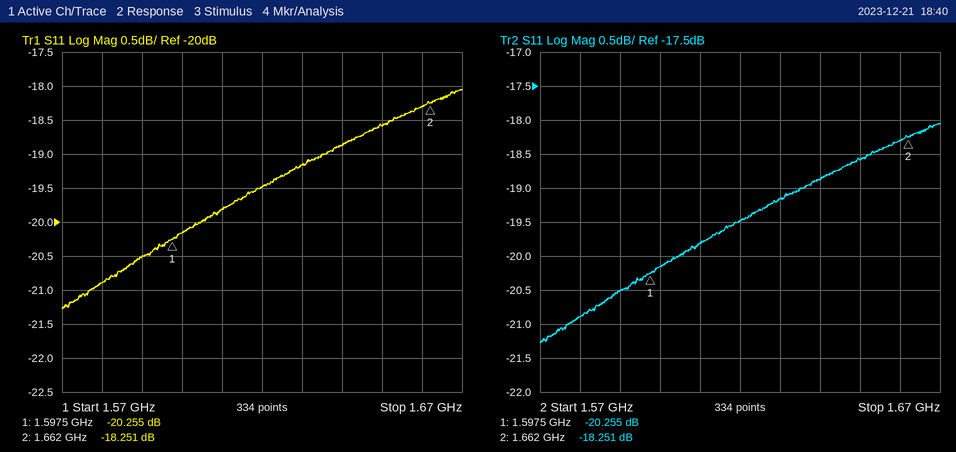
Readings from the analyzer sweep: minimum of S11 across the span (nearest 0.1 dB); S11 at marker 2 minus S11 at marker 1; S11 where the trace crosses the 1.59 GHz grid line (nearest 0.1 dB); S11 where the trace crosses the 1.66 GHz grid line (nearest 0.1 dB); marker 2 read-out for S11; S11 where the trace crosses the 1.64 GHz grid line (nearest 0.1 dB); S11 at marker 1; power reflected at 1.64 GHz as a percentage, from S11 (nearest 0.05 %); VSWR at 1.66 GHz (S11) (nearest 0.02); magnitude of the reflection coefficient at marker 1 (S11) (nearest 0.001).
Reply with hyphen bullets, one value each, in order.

- -21.3 dB
- 2.004 dB
- -20.5 dB
- -18.3 dB
- -18.251 dB
- -18.9 dB
- -20.255 dB
- 1.30 %
- 1.28
- 0.097
